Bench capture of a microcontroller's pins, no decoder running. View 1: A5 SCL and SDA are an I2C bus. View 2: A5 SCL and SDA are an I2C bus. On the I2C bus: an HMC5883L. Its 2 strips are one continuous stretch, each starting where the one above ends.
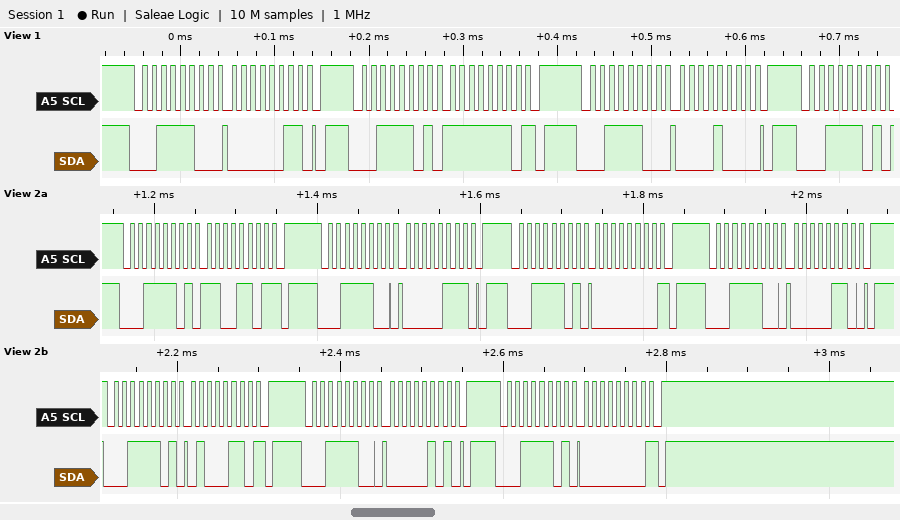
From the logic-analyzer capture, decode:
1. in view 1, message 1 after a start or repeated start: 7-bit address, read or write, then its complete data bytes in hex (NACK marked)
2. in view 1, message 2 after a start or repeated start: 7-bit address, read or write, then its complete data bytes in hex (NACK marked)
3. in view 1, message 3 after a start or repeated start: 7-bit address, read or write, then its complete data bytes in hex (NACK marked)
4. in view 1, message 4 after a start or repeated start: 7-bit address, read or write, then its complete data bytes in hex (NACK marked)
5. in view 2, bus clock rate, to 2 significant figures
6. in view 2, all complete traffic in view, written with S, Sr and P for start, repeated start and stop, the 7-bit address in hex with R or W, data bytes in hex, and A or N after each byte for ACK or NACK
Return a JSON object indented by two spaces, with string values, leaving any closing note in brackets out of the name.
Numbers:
{
  "in view 1, message 1 after a start or repeated start: 7-bit address, read or write, then its complete data bytes in hex": "0x1E write: 03",
  "in view 1, message 2 after a start or repeated start: 7-bit address, read or write, then its complete data bytes in hex": "0x1E read: FE NACK",
  "in view 1, message 3 after a start or repeated start: 7-bit address, read or write, then its complete data bytes in hex": "0x1E write: 08",
  "in view 1, message 4 after a start or repeated start: 7-bit address, read or write, then its complete data bytes in hex": "0x1E read",
  "in view 2, bus clock rate, to 2 significant figures": "100 kHz",
  "in view 2, all complete traffic in view, written with S, Sr and P for start, repeated start and stop, the 7-bit address in hex with R or W, data bytes in hex, and A or N after each byte for ACK or NACK": "S 1ER A CD N P S 1EW A 07 A P S 1ER A 00 N P S 1EW A 06 A P S 1ER A 46 N P S 1EW A 05 A P S 1ER A 00 N P"
}
